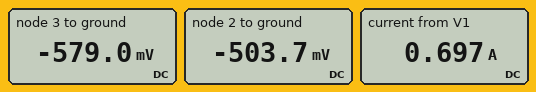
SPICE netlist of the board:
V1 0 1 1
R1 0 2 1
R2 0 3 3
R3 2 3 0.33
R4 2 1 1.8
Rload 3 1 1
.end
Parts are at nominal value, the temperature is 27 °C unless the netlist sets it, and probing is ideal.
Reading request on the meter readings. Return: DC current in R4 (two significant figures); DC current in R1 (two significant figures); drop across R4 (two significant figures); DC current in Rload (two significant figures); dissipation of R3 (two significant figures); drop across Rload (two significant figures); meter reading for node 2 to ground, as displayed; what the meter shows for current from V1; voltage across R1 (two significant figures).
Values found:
280 mA
500 mA
500 mV
420 mA
17 mW
420 mV
-503.7 mV
0.697 A
500 mV
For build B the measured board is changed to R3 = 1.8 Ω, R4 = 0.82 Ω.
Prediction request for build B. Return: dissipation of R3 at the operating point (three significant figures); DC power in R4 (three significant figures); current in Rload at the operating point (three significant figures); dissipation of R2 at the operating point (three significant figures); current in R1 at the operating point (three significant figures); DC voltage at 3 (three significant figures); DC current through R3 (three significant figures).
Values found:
8.04 mW
216 mW
300 mA
163 mW
580 mA
-700 mV
66.8 mA
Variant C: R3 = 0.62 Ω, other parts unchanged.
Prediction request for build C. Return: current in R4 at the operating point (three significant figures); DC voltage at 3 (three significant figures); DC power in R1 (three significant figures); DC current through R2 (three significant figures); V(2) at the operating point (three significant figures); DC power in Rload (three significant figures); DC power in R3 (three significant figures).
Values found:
287 mA
-604 mV
233 mW
201 mA
-483 mV
157 mW
23.6 mW
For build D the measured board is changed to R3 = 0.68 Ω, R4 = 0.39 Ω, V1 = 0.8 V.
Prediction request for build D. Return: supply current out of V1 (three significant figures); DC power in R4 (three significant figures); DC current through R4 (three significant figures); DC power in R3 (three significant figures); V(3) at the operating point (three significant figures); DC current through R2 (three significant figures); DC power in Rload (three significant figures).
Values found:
776 mA
125 mW
565 mA
139 µW
-589 mV
196 mA
44.4 mW
